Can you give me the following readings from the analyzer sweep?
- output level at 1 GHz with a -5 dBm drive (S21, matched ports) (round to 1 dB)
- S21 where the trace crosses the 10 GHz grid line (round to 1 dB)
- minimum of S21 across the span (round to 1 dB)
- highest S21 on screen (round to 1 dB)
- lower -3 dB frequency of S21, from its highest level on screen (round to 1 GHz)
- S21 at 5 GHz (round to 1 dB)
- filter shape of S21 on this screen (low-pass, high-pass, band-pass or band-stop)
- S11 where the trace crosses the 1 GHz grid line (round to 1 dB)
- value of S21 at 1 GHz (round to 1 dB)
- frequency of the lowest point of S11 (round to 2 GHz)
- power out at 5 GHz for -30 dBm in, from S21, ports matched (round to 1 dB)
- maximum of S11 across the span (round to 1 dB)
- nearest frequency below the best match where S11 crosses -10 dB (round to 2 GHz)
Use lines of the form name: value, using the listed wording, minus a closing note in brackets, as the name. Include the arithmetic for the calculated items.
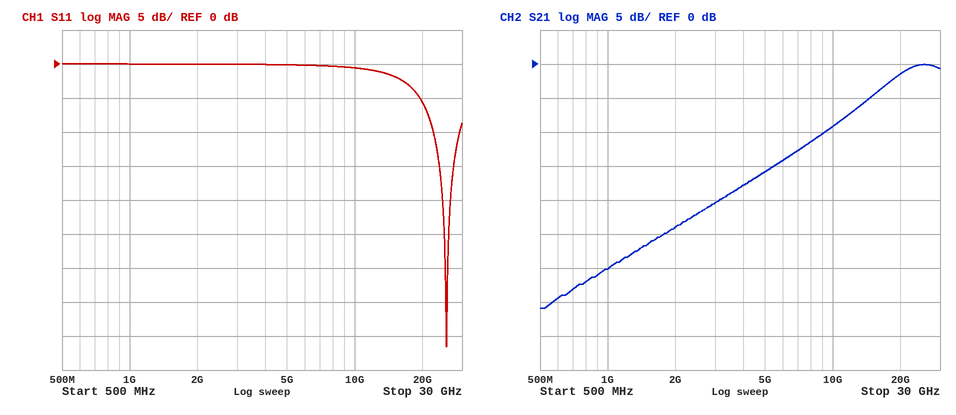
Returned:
output level at 1 GHz with a -5 dBm drive (S21, matched ports): -5 dBm + (-30 dB) = -35 dBm
S21 where the trace crosses the 10 GHz grid line: -9 dB
minimum of S21 across the span: -36 dB
highest S21 on screen: 0 dB
lower -3 dB frequency of S21, from its highest level on screen: 17 GHz
S21 at 5 GHz: -16 dB
filter shape of S21 on this screen: high-pass
S11 where the trace crosses the 1 GHz grid line: 0 dB
value of S21 at 1 GHz: -30 dB
frequency of the lowest point of S11: 26 GHz
power out at 5 GHz for -30 dBm in, from S21, ports matched: -30 dBm + (-16 dB) = -46 dBm
maximum of S11 across the span: 0 dB
nearest frequency below the best match where S11 crosses -10 dB: 22 GHz
